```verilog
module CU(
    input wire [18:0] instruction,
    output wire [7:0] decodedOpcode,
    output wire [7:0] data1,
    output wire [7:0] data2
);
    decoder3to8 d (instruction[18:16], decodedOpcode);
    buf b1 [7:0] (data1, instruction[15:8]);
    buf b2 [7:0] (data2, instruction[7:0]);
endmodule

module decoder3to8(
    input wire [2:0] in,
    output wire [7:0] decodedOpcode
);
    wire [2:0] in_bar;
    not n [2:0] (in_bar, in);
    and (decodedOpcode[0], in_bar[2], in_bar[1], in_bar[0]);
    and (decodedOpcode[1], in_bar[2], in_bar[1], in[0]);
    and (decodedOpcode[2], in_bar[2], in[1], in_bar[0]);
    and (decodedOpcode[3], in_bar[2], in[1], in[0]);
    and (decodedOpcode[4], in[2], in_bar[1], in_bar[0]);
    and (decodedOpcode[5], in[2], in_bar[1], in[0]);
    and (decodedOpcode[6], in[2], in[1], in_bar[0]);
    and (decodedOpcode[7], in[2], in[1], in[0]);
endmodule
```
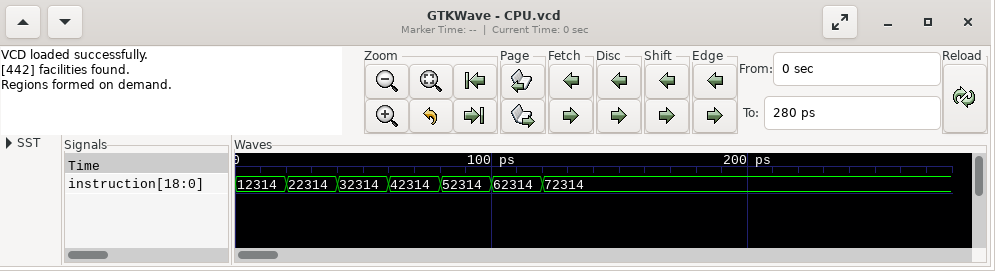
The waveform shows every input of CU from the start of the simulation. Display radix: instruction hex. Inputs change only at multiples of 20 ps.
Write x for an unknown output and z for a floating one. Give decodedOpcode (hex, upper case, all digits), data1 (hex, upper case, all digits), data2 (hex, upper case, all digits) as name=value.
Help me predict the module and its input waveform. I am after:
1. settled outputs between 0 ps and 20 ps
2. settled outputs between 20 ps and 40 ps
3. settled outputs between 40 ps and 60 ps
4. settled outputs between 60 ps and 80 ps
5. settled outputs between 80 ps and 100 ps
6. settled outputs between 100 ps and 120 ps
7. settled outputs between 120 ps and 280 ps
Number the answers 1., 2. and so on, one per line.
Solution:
1. decodedOpcode=02, data1=23, data2=14
2. decodedOpcode=04, data1=23, data2=14
3. decodedOpcode=08, data1=23, data2=14
4. decodedOpcode=10, data1=23, data2=14
5. decodedOpcode=20, data1=23, data2=14
6. decodedOpcode=40, data1=23, data2=14
7. decodedOpcode=80, data1=23, data2=14
